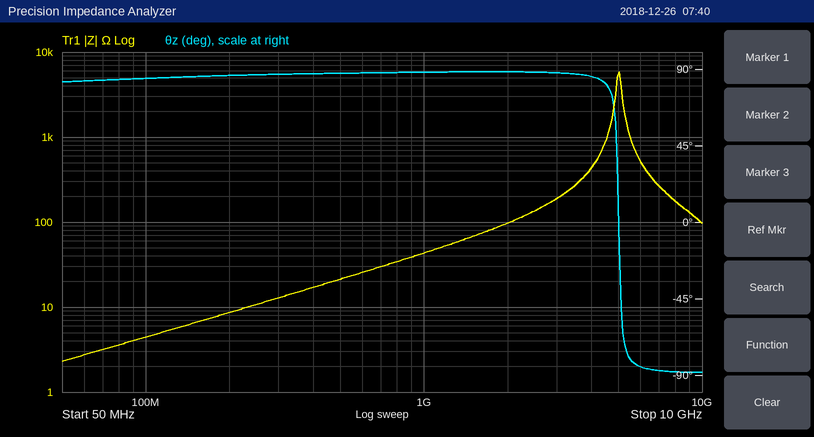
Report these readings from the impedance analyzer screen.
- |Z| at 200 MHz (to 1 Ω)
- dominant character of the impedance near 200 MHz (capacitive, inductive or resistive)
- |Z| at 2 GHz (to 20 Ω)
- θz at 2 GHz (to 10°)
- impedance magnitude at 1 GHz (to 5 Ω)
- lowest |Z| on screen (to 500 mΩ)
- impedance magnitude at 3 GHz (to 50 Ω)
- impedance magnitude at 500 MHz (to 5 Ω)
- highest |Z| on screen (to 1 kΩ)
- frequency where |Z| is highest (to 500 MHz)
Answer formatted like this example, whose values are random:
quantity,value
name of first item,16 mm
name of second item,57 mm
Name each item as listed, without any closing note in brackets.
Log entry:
quantity,value
|Z| at 200 MHz,9 Ω
dominant character of the impedance near 200 MHz,inductive
|Z| at 2 GHz,100 Ω
θz at 2 GHz,90°
impedance magnitude at 1 GHz,45 Ω
lowest |Z| on screen,2.5 Ω
impedance magnitude at 3 GHz,200 Ω
impedance magnitude at 500 MHz,20 Ω
highest |Z| on screen,6 kΩ
frequency where |Z| is highest,5.0 GHz
